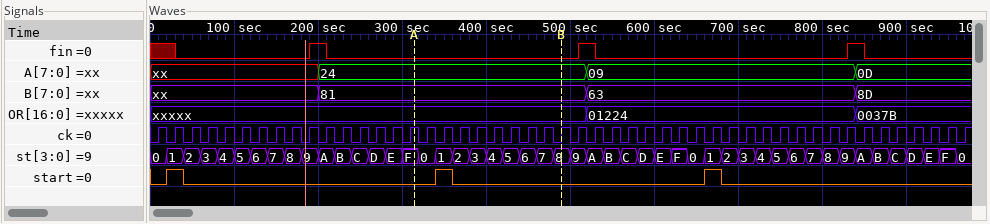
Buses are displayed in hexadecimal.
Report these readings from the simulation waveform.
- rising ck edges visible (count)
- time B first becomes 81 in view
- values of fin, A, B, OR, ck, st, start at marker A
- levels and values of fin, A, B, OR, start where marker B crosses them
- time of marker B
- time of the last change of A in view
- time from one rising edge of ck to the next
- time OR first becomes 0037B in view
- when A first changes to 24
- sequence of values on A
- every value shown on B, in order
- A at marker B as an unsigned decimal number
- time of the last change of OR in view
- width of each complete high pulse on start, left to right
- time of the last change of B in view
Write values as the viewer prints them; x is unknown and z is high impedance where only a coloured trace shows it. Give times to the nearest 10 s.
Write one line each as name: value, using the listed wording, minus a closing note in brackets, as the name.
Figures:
rising ck edges visible: 49
time B first becomes 81 in view: 200 s
values of fin, A, B, OR, ck, st, start at marker A: fin=0, A=24, B=81, OR=xxxxx, ck=1, st=F, start=0
levels and values of fin, A, B, OR, start where marker B crosses them: fin=0, A=24, B=81, OR=xxxxx, start=0
time of marker B: 490 s
time of the last change of A in view: 840 s
time from one rising edge of ck to the next: 20 s
time OR first becomes 0037B in view: 840 s
when A first changes to 24: 200 s
sequence of values on A: xx, 24, 09, 0D
every value shown on B, in order: xx, 81, 63, 8D
A at marker B as an unsigned decimal number: 36
time of the last change of OR in view: 840 s
width of each complete high pulse on start, left to right: 20 s, 20 s, 20 s
time of the last change of B in view: 840 s
